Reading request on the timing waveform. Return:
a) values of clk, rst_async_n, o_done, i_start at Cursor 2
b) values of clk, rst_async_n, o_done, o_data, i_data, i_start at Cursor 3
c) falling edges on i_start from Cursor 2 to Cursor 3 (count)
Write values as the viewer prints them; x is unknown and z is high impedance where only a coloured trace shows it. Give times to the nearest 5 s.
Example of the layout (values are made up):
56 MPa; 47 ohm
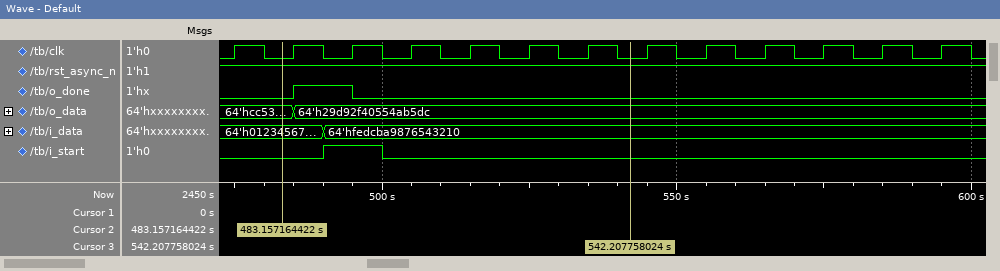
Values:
clk=0, rst_async_n=1, o_done=0, i_start=0; clk=0, rst_async_n=1, o_done=0, o_data=64'h29d92f40554ab5dc, i_data=64'hfedcba9876543210, i_start=0; 1
